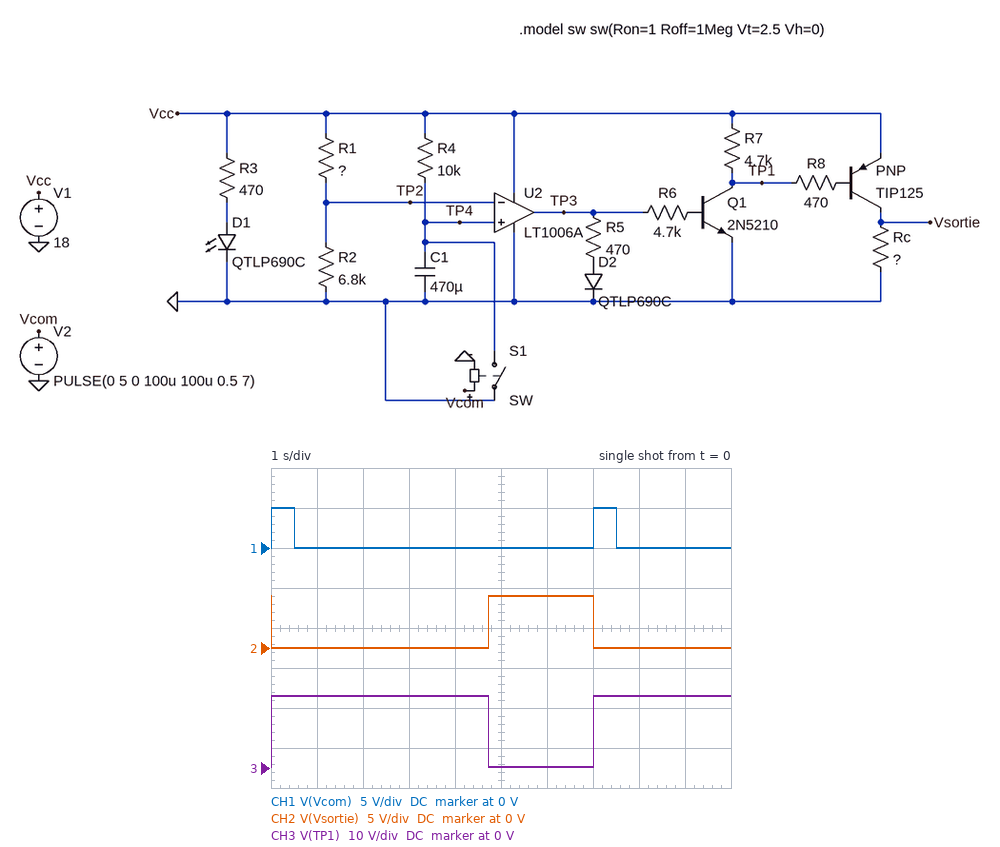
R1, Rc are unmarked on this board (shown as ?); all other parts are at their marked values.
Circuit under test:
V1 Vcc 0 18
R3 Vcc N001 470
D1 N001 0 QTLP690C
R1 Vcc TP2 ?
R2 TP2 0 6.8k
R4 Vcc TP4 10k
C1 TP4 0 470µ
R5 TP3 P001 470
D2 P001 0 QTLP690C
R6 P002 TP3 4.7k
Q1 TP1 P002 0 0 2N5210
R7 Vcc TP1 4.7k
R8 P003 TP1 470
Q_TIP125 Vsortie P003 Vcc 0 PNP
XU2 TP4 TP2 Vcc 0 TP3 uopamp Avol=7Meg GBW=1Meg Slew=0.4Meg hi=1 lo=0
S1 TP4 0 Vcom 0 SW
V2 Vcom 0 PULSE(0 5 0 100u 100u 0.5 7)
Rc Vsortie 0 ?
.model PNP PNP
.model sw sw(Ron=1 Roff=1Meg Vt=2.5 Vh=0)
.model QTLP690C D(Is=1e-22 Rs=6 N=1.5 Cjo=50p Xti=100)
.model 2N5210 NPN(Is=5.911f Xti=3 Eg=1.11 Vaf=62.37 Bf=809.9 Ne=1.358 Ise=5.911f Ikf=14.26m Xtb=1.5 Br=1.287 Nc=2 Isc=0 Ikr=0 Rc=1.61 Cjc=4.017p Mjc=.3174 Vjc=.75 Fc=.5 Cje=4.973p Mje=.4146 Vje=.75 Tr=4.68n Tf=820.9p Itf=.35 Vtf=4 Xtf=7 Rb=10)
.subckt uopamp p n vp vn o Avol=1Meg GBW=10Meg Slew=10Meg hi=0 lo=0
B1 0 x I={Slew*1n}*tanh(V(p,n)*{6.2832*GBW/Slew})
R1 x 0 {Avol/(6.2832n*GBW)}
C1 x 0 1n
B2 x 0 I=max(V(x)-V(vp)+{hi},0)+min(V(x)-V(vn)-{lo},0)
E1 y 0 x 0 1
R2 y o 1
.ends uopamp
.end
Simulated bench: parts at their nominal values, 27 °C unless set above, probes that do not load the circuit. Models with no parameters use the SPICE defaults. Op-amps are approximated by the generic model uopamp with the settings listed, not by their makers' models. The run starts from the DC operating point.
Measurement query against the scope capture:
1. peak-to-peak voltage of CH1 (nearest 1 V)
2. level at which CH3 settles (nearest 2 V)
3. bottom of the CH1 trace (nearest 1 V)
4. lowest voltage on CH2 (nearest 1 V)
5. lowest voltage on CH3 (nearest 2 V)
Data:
5 V
18 V
0 V
0 V
0 V
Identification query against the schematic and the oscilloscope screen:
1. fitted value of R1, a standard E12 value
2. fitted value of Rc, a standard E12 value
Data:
4.7 kΩ
1.8 Ω
